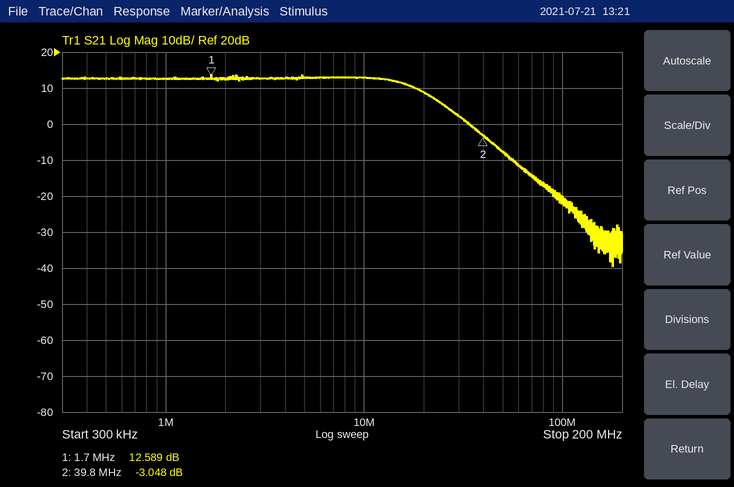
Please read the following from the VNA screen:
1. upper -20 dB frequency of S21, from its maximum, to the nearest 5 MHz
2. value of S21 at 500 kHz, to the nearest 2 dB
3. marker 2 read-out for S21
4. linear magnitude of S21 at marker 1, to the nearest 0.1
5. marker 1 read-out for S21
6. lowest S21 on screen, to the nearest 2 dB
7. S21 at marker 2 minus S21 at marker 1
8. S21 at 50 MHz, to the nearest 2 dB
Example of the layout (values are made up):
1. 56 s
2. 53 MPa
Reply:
1. 45 MHz
2. 12 dB
3. -3.048 dB
4. 4.3
5. 12.589 dB
6. -40 dB
7. -15.637 dB
8. -8 dB
